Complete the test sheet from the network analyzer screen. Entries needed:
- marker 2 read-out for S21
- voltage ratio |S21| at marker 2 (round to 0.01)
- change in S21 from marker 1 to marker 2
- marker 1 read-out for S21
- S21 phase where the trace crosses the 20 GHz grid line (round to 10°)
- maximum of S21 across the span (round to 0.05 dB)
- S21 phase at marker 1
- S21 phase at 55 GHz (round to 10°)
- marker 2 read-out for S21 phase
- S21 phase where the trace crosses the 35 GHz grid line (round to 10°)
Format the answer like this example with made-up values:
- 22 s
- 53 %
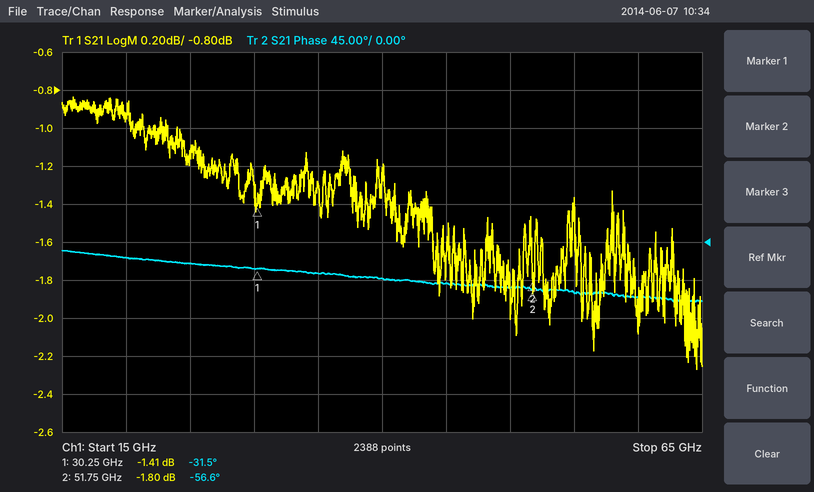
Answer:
- -1.80 dB
- 0.81
- -0.39 dB
- -1.41 dB
- -20°
- -0.85 dB
- -31.5°
- -60°
- -56.6°
- -40°
